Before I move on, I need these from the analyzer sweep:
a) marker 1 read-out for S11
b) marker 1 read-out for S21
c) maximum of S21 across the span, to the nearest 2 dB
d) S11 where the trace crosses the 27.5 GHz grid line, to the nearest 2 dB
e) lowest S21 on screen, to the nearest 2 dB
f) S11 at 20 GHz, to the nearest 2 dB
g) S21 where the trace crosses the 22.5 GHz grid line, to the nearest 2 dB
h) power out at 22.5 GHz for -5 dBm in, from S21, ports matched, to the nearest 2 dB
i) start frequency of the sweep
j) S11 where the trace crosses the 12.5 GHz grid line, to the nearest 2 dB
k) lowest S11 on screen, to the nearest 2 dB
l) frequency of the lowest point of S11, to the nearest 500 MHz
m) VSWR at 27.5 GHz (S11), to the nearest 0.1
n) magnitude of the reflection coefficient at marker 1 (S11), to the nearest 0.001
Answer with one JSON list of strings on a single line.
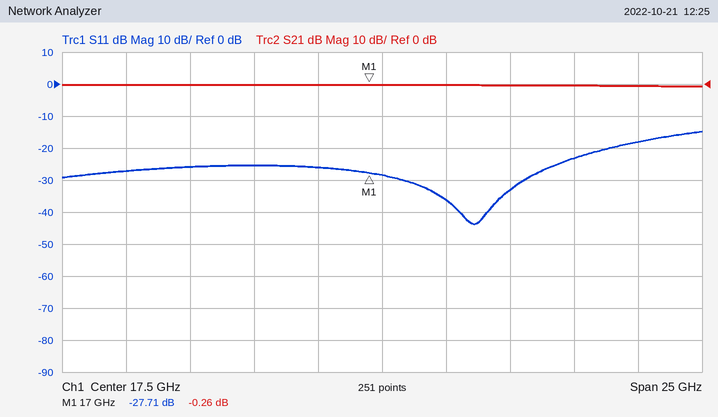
["-27.71 dB", "-0.26 dB", "0 dB", "-18 dB", "0 dB", "-36 dB", "0 dB", "-6 dBm", "5 GHz", "-26 dB", "-44 dB", "21.0 GHz", "1.3", "0.041"]
